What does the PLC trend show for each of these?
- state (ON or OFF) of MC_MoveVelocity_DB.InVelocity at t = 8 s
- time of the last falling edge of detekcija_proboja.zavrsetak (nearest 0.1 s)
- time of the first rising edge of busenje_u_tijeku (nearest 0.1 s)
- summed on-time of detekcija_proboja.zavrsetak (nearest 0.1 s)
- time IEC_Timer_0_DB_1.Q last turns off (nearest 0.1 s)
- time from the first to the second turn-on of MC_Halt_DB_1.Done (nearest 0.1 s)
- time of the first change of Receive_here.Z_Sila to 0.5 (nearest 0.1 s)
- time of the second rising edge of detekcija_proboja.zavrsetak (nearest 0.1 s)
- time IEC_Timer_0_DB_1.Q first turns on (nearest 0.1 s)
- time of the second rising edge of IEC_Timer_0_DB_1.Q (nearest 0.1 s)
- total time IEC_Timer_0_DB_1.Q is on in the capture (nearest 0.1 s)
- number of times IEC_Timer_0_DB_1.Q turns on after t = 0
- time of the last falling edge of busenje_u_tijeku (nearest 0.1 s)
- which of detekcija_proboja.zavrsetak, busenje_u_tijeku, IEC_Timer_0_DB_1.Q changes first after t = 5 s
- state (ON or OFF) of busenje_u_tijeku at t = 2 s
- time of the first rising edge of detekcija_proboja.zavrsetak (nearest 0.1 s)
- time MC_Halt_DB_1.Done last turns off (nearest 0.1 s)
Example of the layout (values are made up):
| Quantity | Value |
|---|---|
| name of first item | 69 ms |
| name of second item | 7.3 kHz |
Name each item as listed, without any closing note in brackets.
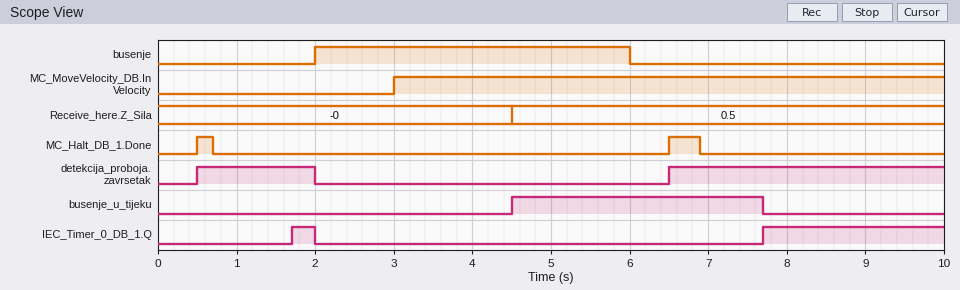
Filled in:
| Quantity | Value |
|---|---|
| state (ON or OFF) of MC_MoveVelocity_DB.InVelocity at t = 8 s | ON |
| time of the last falling edge of detekcija_proboja.zavrsetak | 2.0 s |
| time of the first rising edge of busenje_u_tijeku | 4.5 s |
| summed on-time of detekcija_proboja.zavrsetak | 5.0 s |
| time IEC_Timer_0_DB_1.Q last turns off | 2.0 s |
| time from the first to the second turn-on of MC_Halt_DB_1.Done | 6.0 s |
| time of the first change of Receive_here.Z_Sila to 0.5 | 4.5 s |
| time of the second rising edge of detekcija_proboja.zavrsetak | 6.5 s |
| time IEC_Timer_0_DB_1.Q first turns on | 1.7 s |
| time of the second rising edge of IEC_Timer_0_DB_1.Q | 7.7 s |
| total time IEC_Timer_0_DB_1.Q is on in the capture | 2.6 s |
| number of times IEC_Timer_0_DB_1.Q turns on after t = 0 | 2 |
| time of the last falling edge of busenje_u_tijeku | 7.7 s |
| which of detekcija_proboja.zavrsetak, busenje_u_tijeku, IEC_Timer_0_DB_1.Q changes first after t = 5 s | detekcija_proboja.zavrsetak |
| state (ON or OFF) of busenje_u_tijeku at t = 2 s | OFF |
| time of the first rising edge of detekcija_proboja.zavrsetak | 0.5 s |
| time MC_Halt_DB_1.Done last turns off | 6.9 s |
